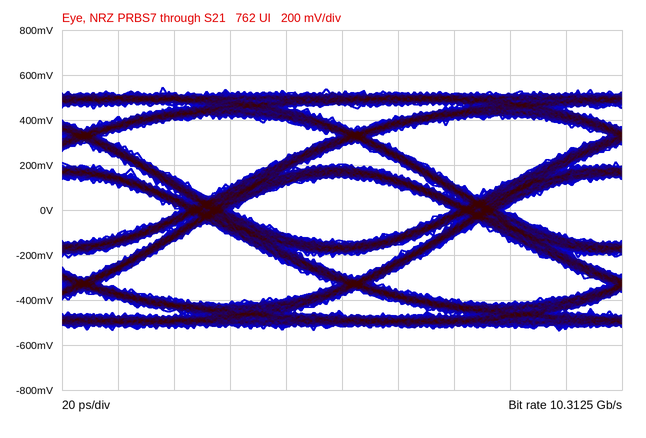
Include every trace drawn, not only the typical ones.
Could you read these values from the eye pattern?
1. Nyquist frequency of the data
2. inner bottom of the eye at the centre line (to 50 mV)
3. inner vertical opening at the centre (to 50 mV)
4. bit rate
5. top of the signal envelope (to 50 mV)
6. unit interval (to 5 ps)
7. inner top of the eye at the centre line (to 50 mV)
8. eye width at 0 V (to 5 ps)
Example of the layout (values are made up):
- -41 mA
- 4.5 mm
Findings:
- 5.15625 GHz
- -150 mV
- 300 mV
- 10.3125 Gb/s
- 550 mV
- 95 ps
- 150 mV
- 80 ps
